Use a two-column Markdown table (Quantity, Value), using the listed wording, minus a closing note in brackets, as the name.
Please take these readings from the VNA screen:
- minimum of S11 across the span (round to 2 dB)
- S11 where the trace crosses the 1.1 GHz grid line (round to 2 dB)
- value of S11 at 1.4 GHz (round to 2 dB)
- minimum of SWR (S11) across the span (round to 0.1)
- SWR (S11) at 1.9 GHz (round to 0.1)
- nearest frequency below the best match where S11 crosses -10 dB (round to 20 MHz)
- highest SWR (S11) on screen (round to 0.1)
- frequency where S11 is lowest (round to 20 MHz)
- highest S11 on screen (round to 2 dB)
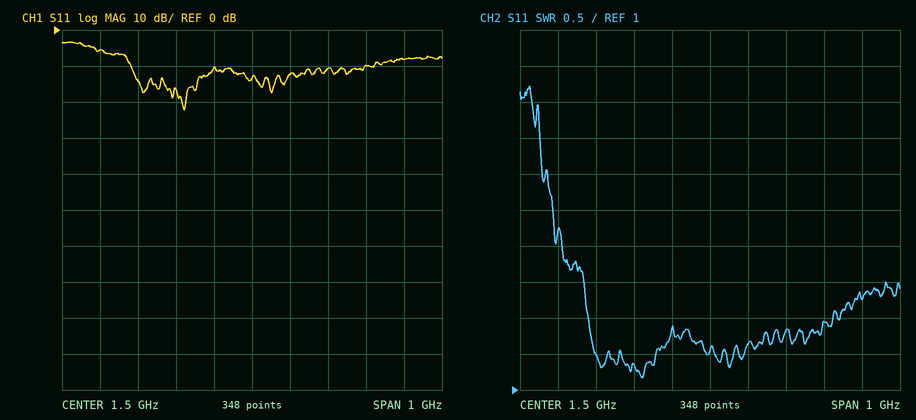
| Quantity | Value |
|---|---|
| minimum of S11 across the span | -22 dB |
| S11 where the trace crosses the 1.1 GHz grid line | -6 dB |
| value of S11 at 1.4 GHz | -10 dB |
| minimum of SWR (S11) across the span | 1.2 |
| SWR (S11) at 1.9 GHz | 2.3 |
| nearest frequency below the best match where S11 crosses -10 dB | 1.18 GHz |
| highest SWR (S11) on screen | 5.2 |
| frequency where S11 is lowest | 1.32 GHz |
| highest S11 on screen | -4 dB |
